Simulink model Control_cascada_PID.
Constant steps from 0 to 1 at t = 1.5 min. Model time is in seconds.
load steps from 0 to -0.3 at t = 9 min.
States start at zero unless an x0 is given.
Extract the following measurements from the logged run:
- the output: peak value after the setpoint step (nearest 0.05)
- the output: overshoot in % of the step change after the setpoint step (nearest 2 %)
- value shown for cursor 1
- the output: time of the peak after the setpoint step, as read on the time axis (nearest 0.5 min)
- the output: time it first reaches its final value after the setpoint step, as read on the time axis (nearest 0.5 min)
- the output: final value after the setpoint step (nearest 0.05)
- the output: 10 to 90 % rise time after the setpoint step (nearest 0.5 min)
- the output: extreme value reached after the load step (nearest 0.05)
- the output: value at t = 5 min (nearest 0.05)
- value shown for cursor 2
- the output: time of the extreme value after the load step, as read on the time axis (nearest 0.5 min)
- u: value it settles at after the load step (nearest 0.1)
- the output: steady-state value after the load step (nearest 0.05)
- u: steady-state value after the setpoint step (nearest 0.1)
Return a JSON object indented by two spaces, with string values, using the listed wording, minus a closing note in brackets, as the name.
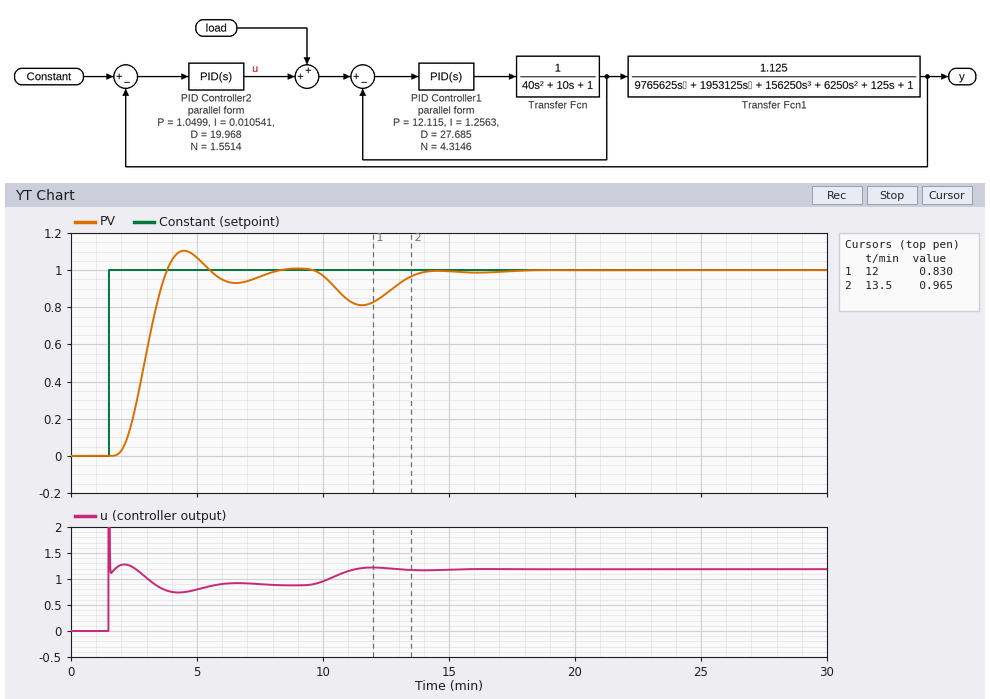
{
  "the output: peak value after the setpoint step": "1.10",
  "the output: overshoot in % of the step change after the setpoint step": "10 %",
  "value shown for cursor 1": "0.830",
  "the output: time of the peak after the setpoint step, as read on the time axis": "4.5 min",
  "the output: time it first reaches its final value after the setpoint step, as read on the time axis": "4.0 min",
  "the output: final value after the setpoint step": "1.00",
  "the output: 10 to 90 % rise time after the setpoint step": "1.5 min",
  "the output: extreme value reached after the load step": "0.80",
  "the output: value at t = 5 min": "1.05",
  "value shown for cursor 2": "0.965",
  "the output: time of the extreme value after the load step, as read on the time axis": "11.5 min",
  "u: value it settles at after the load step": "1.2",
  "the output: steady-state value after the load step": "1.00",
  "u: steady-state value after the setpoint step": "0.9"
}
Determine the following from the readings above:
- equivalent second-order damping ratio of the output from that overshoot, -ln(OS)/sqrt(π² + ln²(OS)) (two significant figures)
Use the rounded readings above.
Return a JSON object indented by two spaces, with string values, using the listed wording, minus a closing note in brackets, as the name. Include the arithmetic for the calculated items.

{
  "equivalent second-order damping ratio of the output from that overshoot, -ln(OS)/sqrt(π² + ln²(OS))": "ln(0.1) = -2.303; 2.303 / sqrt(9.870 + 5.302) = 0.59"
}
